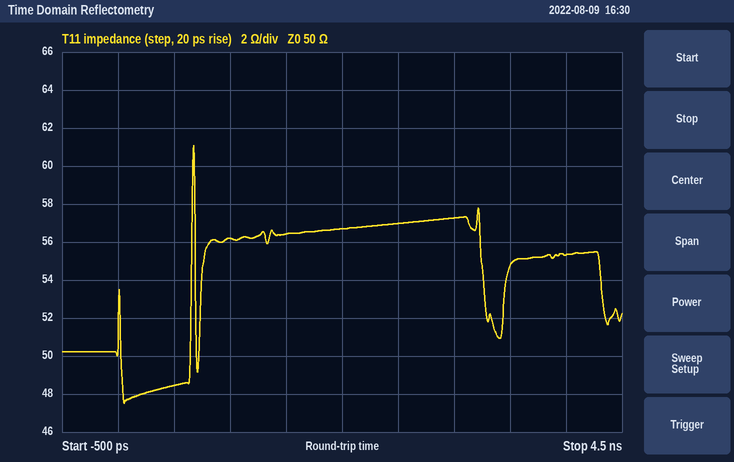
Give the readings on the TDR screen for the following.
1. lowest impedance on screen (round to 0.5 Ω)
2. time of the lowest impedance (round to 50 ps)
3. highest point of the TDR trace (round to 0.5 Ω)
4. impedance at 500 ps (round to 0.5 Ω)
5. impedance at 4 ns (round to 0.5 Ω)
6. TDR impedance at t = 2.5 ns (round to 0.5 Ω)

47.5 Ω
50 ps
61.0 Ω
48.5 Ω
55.5 Ω
57.0 Ω
